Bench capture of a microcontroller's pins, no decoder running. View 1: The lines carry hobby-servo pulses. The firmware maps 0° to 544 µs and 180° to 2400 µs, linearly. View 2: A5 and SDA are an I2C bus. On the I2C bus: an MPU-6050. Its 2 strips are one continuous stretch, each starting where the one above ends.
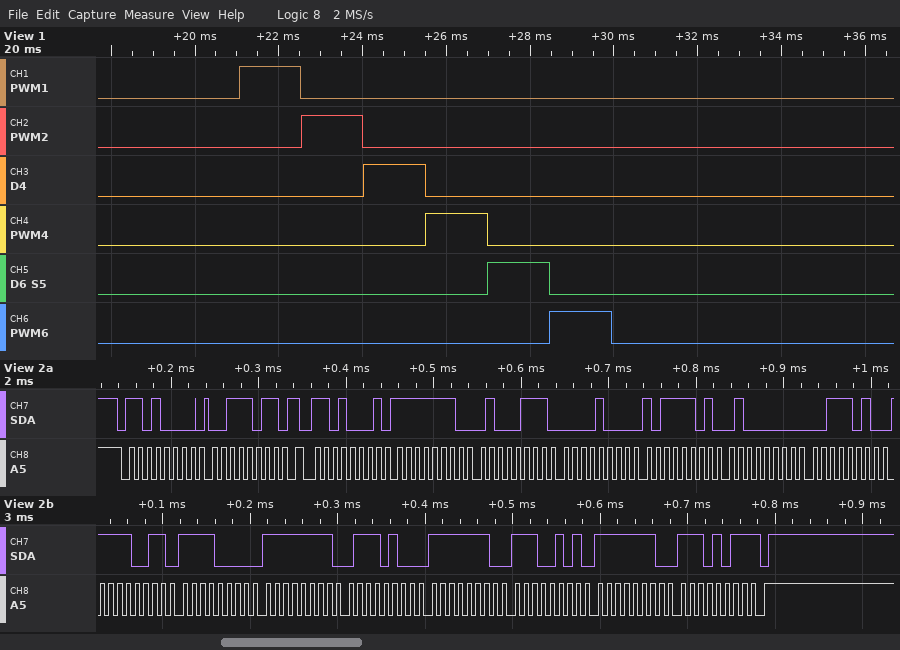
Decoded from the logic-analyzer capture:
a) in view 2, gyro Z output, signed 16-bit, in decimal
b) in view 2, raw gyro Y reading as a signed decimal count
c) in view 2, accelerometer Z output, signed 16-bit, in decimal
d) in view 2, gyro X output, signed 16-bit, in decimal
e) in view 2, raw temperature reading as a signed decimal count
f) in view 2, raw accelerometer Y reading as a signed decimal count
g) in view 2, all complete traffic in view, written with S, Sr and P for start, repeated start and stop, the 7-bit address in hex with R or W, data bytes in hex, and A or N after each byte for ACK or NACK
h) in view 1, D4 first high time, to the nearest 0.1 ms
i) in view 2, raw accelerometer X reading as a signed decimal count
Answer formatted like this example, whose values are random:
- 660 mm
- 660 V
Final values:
- -277
- -283
- 16442
- -140
- -3088
- 2237
- S 68W A 3B A Sr 68R A FE A 47 A 08 A BD A 40 A 3A A F3 A F0 A FF A 74 A FE A E5 A FE A EB N P
- 1.5 ms
- -441
